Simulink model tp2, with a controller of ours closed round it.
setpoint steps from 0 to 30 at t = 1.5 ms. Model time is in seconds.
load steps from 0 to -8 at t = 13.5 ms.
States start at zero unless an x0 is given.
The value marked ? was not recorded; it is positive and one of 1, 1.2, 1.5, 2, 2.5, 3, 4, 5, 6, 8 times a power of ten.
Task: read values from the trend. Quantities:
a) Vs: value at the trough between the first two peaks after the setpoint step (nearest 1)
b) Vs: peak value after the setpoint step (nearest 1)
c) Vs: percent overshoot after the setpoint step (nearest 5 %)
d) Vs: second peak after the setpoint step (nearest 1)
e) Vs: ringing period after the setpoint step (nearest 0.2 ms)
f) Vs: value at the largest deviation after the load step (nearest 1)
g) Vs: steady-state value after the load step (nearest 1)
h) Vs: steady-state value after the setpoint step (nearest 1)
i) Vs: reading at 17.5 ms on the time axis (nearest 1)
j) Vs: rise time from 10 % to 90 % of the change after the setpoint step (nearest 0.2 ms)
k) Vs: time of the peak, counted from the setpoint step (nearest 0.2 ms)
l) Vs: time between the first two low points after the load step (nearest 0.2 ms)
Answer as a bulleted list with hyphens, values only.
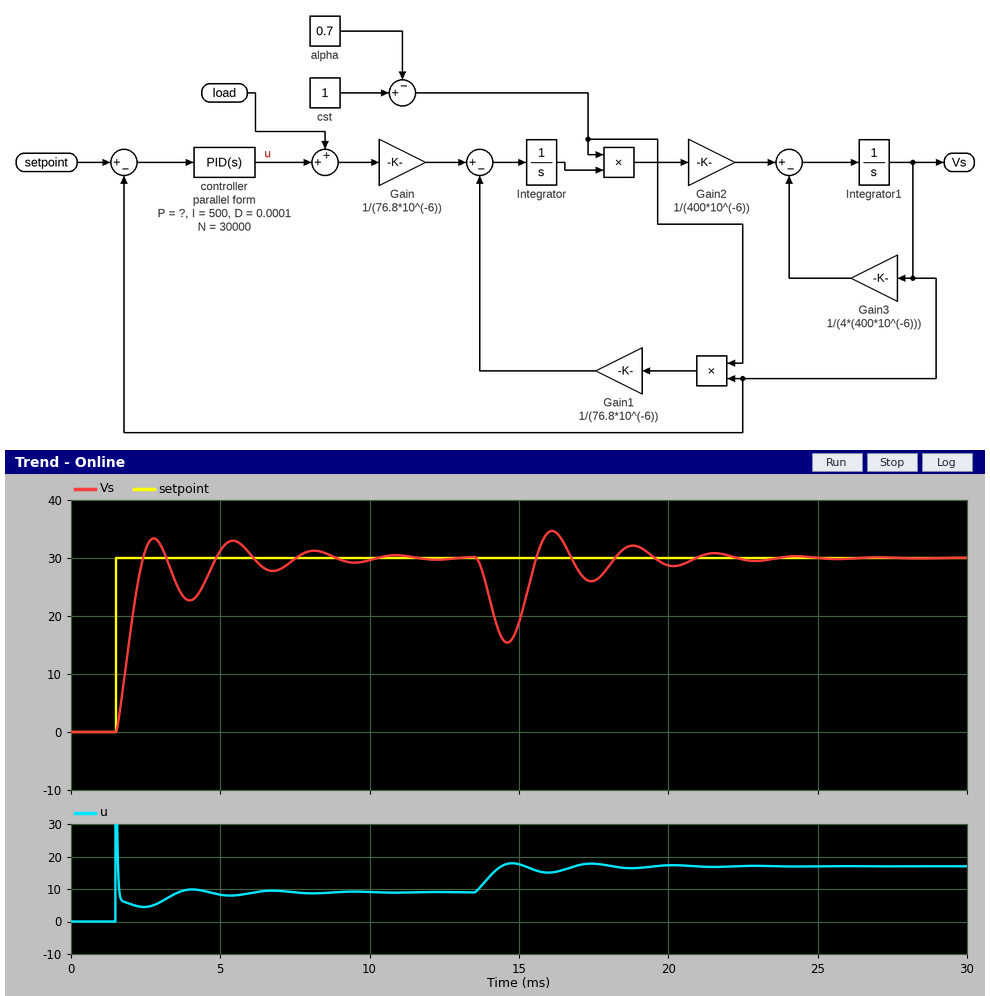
- 23
- 33
- 10 %
- 33
- 2.6 ms
- 15
- 30
- 30
- 26
- 0.6 ms
- 1.2 ms
- 2.8 ms
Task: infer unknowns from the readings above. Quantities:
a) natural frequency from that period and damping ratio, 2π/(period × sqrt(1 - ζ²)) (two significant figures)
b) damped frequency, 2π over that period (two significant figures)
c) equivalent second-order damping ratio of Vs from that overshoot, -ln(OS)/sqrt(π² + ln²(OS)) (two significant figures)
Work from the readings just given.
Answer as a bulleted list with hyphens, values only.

- 3.0 rad/ms
- 2.4 rad/ms
- 0.59
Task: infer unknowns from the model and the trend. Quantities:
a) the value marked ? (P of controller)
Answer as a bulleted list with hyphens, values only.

- 0.3
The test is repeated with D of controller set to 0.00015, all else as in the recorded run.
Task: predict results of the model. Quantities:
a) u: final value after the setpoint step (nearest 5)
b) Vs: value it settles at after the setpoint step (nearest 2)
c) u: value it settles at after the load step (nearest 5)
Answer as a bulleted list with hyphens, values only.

- 10
- 30
- 15
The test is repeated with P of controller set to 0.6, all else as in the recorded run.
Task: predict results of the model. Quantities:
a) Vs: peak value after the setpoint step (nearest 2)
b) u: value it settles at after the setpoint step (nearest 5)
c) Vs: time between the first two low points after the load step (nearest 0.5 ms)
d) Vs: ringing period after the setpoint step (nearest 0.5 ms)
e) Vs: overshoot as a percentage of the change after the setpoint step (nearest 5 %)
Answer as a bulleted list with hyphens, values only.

- 36
- 10
- 2.0 ms
- 2.0 ms
- 20 %
